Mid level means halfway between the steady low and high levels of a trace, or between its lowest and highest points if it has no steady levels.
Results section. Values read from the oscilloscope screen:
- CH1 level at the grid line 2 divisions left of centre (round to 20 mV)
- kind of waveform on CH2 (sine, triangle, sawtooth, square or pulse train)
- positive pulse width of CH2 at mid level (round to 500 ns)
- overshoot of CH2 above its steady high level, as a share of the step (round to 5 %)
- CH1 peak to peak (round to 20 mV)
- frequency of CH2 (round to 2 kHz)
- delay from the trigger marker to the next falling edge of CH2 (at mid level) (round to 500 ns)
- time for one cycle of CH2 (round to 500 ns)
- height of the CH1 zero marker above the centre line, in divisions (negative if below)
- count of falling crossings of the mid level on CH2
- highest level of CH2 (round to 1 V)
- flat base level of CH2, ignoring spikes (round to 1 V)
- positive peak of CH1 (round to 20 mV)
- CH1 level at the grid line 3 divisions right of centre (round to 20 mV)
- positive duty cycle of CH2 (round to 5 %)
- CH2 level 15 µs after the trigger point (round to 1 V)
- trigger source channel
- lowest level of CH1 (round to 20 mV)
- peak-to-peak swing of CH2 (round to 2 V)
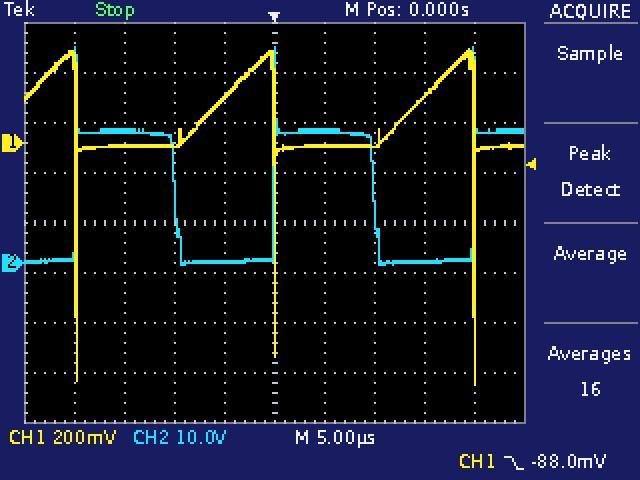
-20 mV
square
10.0 µs
65 %
1.34 V
50 kHz
10.0 µs
20.0 µs
+1.6 div
2
43 V
0 V
380 mV
180 mV
50 %
0 V
CH1
-960 mV
44 V
